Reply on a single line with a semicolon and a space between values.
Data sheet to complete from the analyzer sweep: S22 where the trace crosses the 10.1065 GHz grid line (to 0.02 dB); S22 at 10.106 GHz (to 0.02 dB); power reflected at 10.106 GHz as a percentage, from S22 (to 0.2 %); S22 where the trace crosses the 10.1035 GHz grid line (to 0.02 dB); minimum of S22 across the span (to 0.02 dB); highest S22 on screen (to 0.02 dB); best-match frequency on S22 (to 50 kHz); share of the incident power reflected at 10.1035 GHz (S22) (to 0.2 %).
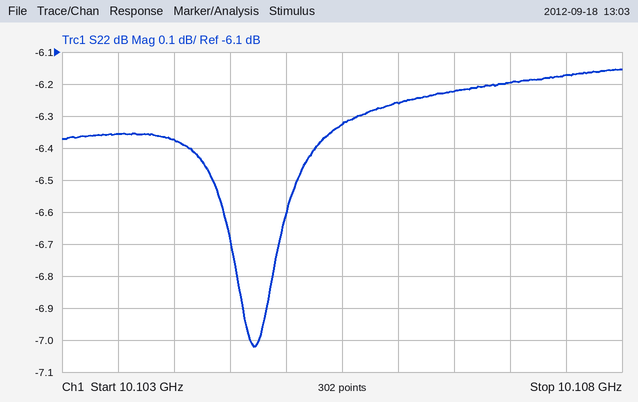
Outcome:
-6.22 dB; -6.26 dB; 23.6 %; -6.36 dB; -7.02 dB; -6.16 dB; 10.10470 GHz; 23.2 %
